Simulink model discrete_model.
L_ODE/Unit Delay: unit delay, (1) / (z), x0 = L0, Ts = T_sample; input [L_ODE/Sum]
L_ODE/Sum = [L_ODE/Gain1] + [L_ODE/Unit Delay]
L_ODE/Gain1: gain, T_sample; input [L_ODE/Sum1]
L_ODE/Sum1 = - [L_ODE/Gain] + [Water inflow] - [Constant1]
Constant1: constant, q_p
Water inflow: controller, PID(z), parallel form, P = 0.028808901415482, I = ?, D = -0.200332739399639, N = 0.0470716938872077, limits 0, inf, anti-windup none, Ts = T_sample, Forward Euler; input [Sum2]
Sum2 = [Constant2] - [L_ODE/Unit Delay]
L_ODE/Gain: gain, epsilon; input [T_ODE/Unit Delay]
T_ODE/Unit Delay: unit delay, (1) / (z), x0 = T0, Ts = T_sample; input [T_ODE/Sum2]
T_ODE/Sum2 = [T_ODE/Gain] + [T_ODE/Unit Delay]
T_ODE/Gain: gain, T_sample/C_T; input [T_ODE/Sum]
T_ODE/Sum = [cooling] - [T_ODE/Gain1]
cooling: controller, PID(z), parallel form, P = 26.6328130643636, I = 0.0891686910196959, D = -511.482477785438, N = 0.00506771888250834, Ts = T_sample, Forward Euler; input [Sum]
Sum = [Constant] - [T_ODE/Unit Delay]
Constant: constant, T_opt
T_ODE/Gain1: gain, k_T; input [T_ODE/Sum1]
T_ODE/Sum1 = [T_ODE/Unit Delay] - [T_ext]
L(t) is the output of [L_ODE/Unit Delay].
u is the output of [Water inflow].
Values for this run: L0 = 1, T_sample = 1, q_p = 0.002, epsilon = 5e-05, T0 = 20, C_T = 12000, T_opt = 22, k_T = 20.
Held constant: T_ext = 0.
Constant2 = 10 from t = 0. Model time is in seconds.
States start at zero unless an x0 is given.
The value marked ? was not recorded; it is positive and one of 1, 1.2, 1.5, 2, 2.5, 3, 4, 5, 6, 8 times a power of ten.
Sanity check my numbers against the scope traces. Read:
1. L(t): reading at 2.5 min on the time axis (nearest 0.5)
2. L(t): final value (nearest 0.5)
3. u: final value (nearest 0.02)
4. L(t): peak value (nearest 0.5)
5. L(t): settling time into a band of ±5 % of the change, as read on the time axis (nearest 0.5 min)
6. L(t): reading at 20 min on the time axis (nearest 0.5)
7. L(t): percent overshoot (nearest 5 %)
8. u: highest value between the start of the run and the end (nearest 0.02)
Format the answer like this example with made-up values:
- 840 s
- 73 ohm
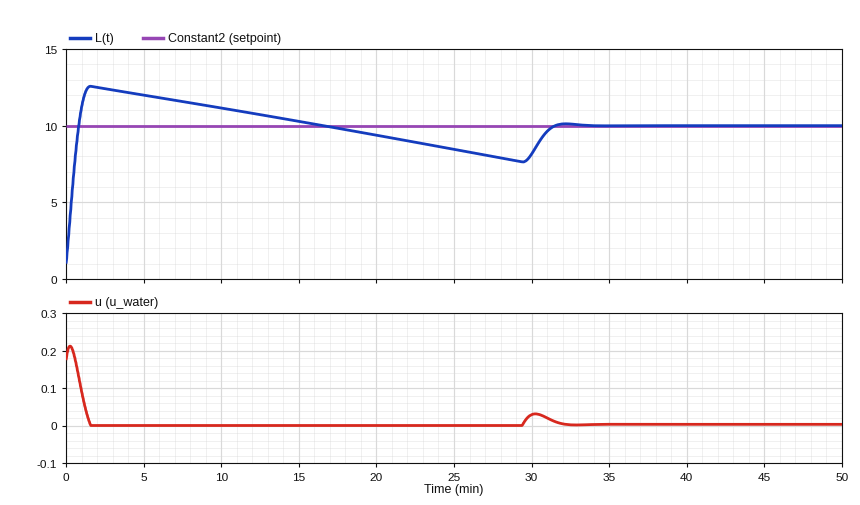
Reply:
- 12.5
- 10.0
- 0.00
- 12.5
- 31.0 min
- 9.5
- 30 %
- 0.22
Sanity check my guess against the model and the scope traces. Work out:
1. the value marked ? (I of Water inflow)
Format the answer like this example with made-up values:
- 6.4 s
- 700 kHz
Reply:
- 0.0005
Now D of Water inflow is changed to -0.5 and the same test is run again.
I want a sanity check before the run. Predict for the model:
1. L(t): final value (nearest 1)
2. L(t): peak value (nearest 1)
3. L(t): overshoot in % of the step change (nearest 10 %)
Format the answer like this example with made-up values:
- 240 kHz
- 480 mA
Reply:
- 10
- 14
- 40 %
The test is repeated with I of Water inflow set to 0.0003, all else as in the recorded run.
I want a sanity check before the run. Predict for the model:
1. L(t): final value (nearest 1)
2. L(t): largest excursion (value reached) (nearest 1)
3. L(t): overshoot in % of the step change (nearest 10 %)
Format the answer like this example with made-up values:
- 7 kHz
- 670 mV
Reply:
- 10
- 12
- 20 %
